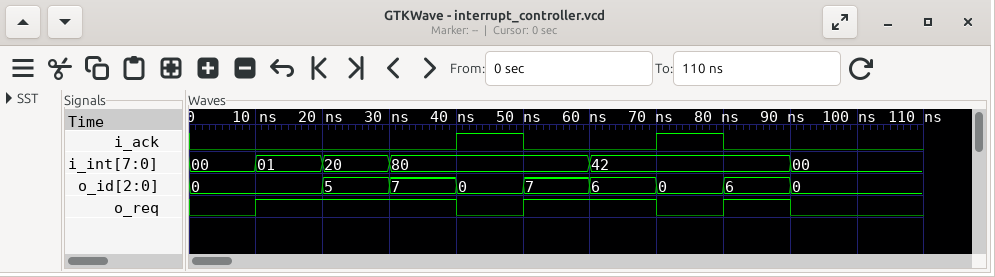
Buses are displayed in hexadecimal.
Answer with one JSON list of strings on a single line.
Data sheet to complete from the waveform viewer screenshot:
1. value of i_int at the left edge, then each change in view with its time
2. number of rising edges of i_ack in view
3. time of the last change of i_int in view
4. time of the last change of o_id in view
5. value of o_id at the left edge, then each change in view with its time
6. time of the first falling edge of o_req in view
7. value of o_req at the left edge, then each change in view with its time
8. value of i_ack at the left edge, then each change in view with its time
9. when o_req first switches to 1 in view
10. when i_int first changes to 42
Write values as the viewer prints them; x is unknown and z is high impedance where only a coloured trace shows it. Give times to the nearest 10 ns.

["00, 01 at 10 ns, 20 at 20 ns, 80 at 30 ns, 42 at 60 ns, 00 at 90 ns", "2", "90 ns", "90 ns", "0, 5 at 20 ns, 7 at 30 ns, 0 at 40 ns, 7 at 50 ns, 6 at 60 ns, 0 at 70 ns, 6 at 80 ns, 0 at 90 ns", "40 ns", "0, 1 at 10 ns, 0 at 40 ns, 1 at 50 ns, 0 at 70 ns, 1 at 80 ns, 0 at 90 ns", "0, 1 at 40 ns, 0 at 50 ns, 1 at 70 ns, 0 at 80 ns", "10 ns", "60 ns"]
